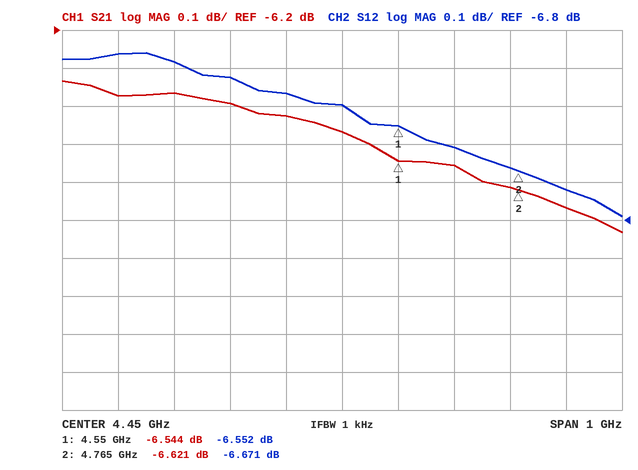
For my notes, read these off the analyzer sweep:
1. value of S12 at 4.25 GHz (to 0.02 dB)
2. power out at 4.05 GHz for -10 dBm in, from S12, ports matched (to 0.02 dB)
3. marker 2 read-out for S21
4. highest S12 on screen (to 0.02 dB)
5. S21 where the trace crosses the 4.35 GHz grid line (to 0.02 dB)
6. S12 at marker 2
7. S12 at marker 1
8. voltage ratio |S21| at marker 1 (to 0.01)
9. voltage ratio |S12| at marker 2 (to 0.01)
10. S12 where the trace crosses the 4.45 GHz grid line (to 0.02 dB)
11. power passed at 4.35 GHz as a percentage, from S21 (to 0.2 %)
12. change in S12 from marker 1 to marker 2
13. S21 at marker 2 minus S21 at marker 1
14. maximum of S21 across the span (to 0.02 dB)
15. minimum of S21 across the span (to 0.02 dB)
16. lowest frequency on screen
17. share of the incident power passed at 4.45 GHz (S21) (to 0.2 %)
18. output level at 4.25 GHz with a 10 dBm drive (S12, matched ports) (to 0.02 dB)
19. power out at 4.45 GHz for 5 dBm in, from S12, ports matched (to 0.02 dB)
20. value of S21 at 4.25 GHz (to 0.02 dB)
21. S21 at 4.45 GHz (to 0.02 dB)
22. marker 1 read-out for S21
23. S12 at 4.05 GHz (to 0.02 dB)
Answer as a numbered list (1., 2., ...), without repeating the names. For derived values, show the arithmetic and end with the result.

1. -6.42 dB
2. -10 dBm + (-6.36 dB) = -16.36 dBm
3. -6.621 dB
4. -6.36 dB
5. -6.42 dB
6. -6.671 dB
7. -6.552 dB
8. 10^(-6.544/20) ≈ 0.47
9. 10^(-6.671/20) ≈ 0.46
10. -6.50 dB
11. 10^(-6.42/10) ≈ 22.8 %
12. -6.671 − (-6.552) = -0.119 dB
13. -6.621 − (-6.544) = -0.077 dB
14. -6.34 dB
15. -6.74 dB
16. 3.95 GHz
17. 10^(-6.46/10) ≈ 22.6 %
18. 10 dBm + (-6.42 dB) = 3.58 dBm
19. 5 dBm + (-6.50 dB) = -1.50 dBm
20. -6.40 dB
21. -6.46 dB
22. -6.544 dB
23. -6.36 dB
